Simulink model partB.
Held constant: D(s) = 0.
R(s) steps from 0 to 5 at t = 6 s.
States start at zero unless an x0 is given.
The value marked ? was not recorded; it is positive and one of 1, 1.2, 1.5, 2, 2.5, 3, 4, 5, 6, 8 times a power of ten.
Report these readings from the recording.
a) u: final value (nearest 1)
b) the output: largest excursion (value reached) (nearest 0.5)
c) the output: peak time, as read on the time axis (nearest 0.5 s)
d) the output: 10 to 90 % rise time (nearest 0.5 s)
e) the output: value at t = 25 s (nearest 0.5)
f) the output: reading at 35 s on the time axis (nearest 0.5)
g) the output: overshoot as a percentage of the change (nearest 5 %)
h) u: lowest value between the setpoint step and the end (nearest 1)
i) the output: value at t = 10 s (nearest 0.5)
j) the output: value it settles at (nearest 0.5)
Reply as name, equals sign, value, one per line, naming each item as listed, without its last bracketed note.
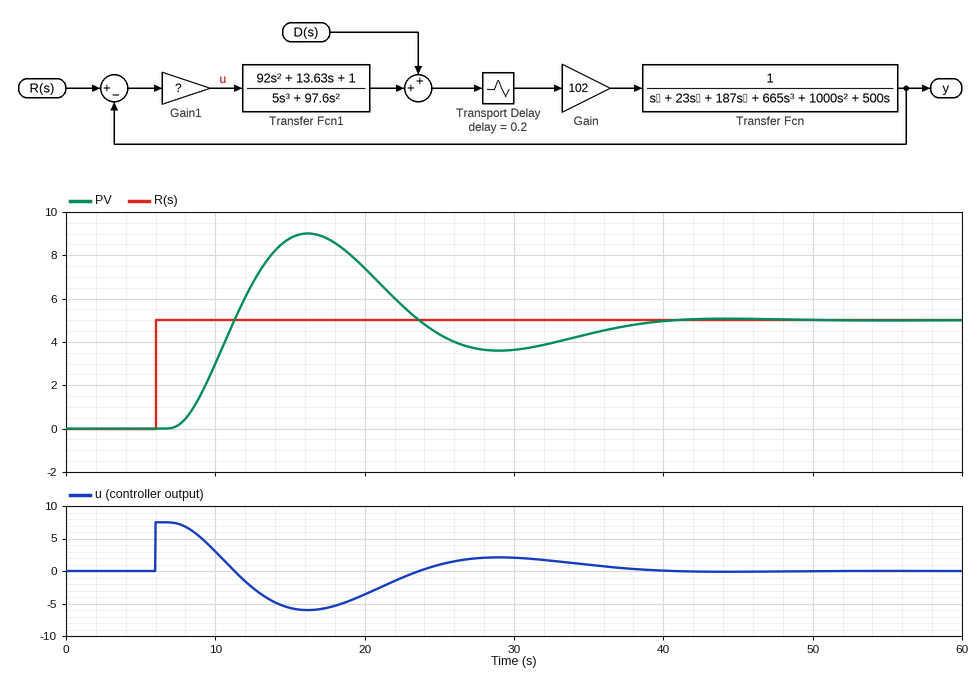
u: final value = 0
the output: largest excursion (value reached) = 9.0
the output: peak time, as read on the time axis = 16.0 s
the output: 10 to 90 % rise time = 3.0 s
the output: value at t = 25 s = 4.5
the output: reading at 35 s on the time axis = 4.5
the output: overshoot as a percentage of the change = 80 %
u: lowest value between the setpoint step and the end = -6
the output: value at t = 10 s = 3.0
the output: value it settles at = 5.0
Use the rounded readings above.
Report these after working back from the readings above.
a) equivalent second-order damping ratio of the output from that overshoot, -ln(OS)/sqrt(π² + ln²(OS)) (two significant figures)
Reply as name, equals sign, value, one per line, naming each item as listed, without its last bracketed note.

equivalent second-order damping ratio of the output from that overshoot, -ln(OS)/sqrt(π² + ln²(OS)) = 0.071
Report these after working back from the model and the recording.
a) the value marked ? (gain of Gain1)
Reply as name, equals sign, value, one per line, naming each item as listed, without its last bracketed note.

the value marked ? = 1.5
